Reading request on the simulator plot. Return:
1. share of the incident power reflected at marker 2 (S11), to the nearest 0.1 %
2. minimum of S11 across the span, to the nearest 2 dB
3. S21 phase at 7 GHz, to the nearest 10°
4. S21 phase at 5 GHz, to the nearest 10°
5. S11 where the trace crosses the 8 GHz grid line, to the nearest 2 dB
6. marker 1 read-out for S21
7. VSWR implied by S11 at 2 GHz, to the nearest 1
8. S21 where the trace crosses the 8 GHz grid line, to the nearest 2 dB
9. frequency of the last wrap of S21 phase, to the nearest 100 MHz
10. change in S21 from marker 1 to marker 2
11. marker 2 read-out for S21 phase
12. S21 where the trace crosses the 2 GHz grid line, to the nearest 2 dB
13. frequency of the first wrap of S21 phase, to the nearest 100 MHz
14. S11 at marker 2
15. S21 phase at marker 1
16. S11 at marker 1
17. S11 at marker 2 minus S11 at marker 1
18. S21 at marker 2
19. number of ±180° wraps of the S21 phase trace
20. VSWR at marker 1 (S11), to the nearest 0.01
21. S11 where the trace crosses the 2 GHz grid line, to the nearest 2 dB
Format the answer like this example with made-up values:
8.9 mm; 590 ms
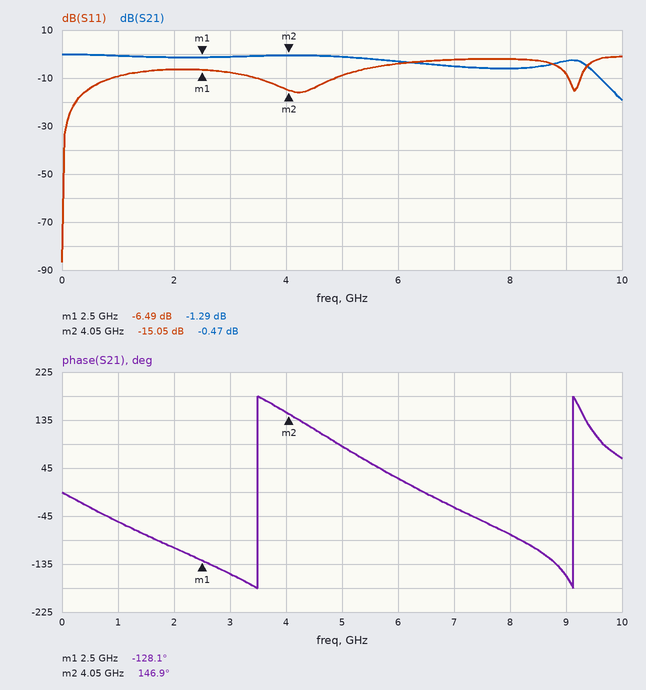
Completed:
3.1 %; -86 dB; -30°; 90°; -2 dB; -1.29 dB; 3; -6 dB; 9.1 GHz; 0.82 dB; 146.9°; -2 dB; 3.5 GHz; -15.05 dB; -128.1°; -6.49 dB; -8.56 dB; -0.47 dB; 2; 2.80; -6 dB
